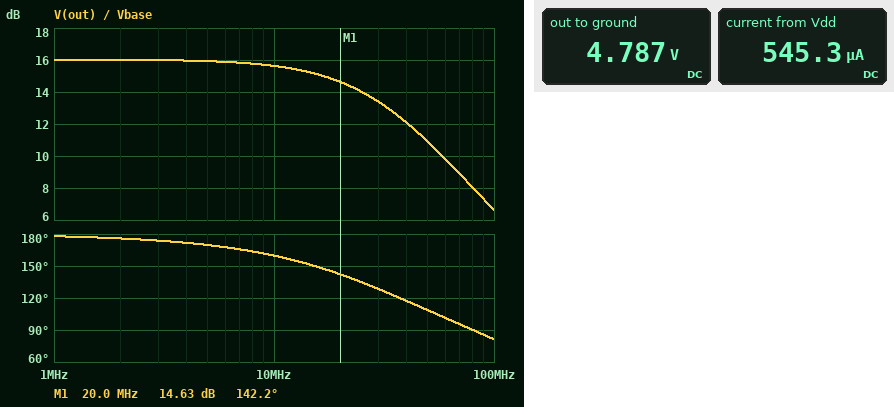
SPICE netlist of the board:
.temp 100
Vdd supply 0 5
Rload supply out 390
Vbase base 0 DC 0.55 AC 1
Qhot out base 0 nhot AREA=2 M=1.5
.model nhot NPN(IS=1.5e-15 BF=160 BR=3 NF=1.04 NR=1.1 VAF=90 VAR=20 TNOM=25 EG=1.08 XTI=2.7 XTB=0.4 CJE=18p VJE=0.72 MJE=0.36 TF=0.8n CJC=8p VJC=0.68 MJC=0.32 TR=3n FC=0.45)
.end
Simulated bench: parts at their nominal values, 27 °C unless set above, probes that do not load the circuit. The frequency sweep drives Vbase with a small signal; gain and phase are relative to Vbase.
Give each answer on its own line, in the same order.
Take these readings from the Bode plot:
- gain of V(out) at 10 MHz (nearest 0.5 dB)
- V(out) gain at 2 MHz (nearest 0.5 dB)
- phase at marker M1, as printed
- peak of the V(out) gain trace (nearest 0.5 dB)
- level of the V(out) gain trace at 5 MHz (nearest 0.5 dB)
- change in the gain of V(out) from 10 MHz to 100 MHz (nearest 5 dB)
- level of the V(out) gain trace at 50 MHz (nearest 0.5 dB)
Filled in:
15.5 dB
16.0 dB
142.2 deg
16.0 dB
16.0 dB
-10 dB
11.0 dB
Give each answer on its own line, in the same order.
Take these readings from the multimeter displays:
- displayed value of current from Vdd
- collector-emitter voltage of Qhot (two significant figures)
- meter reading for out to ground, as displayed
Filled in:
545.3 µA
4.8 V
4.787 V
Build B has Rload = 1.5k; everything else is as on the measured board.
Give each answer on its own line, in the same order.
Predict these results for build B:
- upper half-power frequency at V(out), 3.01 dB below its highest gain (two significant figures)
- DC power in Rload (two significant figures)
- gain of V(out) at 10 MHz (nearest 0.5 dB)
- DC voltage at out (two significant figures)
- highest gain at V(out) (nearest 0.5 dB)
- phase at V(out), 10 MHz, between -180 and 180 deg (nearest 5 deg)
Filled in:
8.0 MHz
440 µW
23.5 dB
4.2 V
27.5 dB
125 deg
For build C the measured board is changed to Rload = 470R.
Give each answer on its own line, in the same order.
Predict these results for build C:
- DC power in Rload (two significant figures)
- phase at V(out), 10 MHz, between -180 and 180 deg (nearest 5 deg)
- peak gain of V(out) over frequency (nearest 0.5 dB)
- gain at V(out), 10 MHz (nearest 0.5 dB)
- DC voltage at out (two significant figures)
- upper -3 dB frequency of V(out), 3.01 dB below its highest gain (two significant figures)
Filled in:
140 µW
155 deg
17.5 dB
17.0 dB
4.7 V
27 MHz
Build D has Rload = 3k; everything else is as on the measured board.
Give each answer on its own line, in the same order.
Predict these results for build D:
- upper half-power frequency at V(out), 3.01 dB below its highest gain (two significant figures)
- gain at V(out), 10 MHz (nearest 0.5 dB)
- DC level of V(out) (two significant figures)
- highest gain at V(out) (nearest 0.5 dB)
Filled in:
3.8 MHz
24.5 dB
3.4 V
33.5 dB
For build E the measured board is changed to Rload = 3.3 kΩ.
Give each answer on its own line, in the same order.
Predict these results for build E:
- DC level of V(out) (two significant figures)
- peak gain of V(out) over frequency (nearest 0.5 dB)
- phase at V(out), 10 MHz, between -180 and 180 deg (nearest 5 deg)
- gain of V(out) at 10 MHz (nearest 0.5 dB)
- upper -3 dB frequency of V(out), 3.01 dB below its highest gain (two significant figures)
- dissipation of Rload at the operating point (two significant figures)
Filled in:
3.2 V
34.5 dB
105 deg
24.5 dB
3.4 MHz
950 µW
